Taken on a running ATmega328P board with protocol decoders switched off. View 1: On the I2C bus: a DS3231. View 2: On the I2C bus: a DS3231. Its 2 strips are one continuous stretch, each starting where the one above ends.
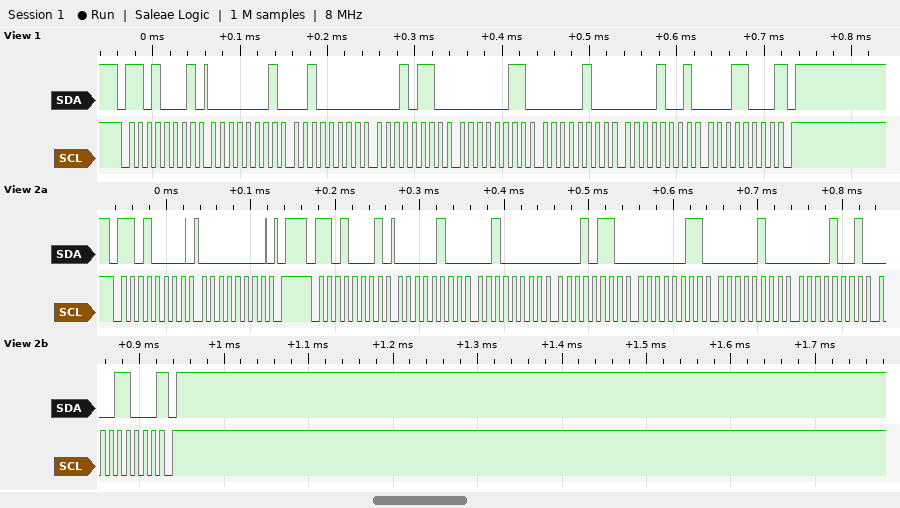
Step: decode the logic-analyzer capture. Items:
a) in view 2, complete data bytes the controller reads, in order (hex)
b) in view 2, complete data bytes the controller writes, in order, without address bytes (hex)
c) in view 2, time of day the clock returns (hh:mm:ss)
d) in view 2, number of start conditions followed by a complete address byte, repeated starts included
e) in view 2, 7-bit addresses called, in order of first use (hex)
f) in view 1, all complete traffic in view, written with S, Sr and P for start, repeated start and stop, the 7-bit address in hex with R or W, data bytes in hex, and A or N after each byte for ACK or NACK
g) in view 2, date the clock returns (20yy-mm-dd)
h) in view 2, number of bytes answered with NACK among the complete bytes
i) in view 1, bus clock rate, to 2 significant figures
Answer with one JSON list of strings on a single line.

["04 20 16 03 04 09 18", "00", "16:20:04", "2", "0x68", "S 68R A 01 A 20 A 16 A 03 A 04 A 09 A 18 N P", "2018-09-04", "1", "100 kHz"]
